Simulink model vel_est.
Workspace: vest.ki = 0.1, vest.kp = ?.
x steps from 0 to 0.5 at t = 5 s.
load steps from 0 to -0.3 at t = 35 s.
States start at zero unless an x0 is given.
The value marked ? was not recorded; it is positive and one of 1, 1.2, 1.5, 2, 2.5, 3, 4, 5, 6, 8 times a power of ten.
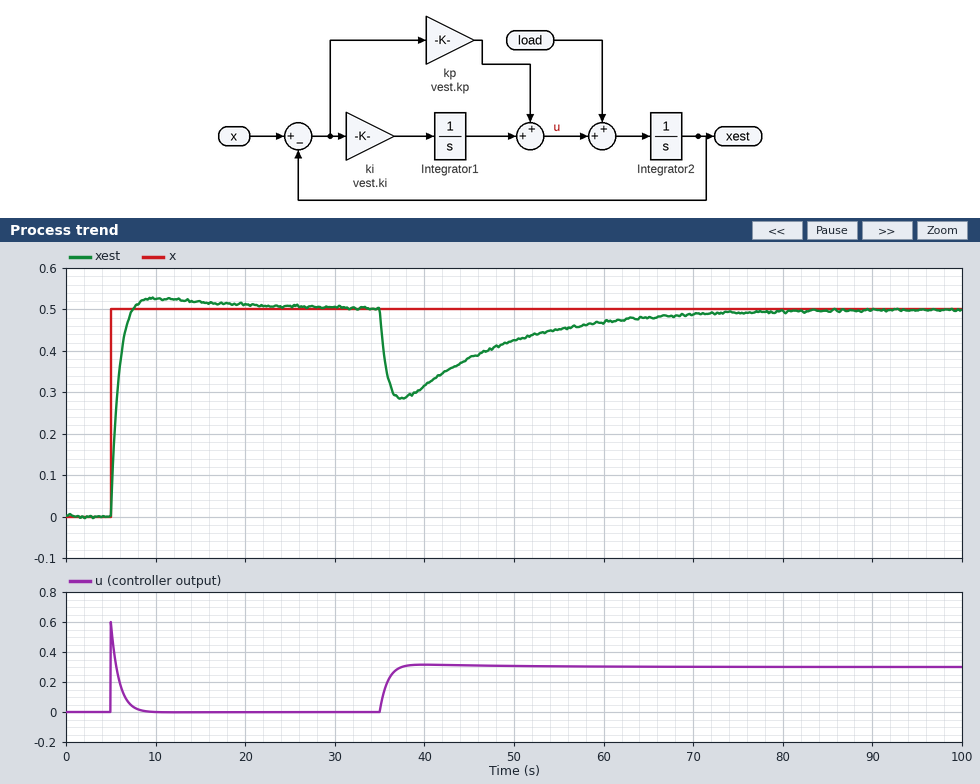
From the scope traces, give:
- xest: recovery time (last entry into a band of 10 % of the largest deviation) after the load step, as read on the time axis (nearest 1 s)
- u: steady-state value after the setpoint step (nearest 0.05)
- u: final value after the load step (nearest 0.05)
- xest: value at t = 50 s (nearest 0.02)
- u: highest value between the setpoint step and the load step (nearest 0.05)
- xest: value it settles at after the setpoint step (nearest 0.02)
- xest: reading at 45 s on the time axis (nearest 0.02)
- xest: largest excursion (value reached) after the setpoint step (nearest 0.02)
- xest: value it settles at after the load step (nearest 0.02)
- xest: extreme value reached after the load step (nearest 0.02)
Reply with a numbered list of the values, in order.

1. 64 s
2. 0.00
3. 0.30
4. 0.42
5. 0.60
6. 0.50
7. 0.38
8. 0.52
9. 0.50
10. 0.28
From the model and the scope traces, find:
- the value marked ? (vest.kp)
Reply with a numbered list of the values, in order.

1. 1.2
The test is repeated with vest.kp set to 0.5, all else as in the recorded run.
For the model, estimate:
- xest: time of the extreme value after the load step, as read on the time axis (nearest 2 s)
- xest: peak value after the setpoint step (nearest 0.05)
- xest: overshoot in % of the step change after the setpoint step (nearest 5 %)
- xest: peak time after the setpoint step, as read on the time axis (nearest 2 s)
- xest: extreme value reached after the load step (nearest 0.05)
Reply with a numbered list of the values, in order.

1. 38 s
2. 0.60
3. 20 %
4. 12 s
5. 0.10
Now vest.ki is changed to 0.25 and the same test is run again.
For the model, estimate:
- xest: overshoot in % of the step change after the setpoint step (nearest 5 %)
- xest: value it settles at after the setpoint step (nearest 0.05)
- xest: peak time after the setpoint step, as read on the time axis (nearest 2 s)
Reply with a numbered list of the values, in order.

1. 10 %
2. 0.50
3. 8 s
